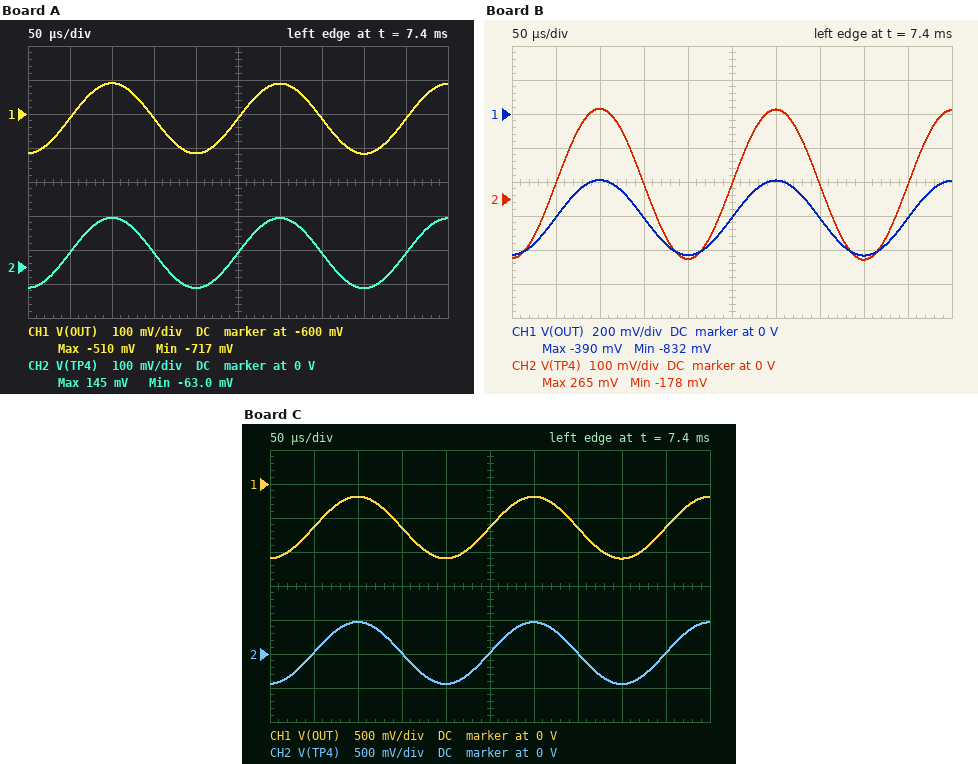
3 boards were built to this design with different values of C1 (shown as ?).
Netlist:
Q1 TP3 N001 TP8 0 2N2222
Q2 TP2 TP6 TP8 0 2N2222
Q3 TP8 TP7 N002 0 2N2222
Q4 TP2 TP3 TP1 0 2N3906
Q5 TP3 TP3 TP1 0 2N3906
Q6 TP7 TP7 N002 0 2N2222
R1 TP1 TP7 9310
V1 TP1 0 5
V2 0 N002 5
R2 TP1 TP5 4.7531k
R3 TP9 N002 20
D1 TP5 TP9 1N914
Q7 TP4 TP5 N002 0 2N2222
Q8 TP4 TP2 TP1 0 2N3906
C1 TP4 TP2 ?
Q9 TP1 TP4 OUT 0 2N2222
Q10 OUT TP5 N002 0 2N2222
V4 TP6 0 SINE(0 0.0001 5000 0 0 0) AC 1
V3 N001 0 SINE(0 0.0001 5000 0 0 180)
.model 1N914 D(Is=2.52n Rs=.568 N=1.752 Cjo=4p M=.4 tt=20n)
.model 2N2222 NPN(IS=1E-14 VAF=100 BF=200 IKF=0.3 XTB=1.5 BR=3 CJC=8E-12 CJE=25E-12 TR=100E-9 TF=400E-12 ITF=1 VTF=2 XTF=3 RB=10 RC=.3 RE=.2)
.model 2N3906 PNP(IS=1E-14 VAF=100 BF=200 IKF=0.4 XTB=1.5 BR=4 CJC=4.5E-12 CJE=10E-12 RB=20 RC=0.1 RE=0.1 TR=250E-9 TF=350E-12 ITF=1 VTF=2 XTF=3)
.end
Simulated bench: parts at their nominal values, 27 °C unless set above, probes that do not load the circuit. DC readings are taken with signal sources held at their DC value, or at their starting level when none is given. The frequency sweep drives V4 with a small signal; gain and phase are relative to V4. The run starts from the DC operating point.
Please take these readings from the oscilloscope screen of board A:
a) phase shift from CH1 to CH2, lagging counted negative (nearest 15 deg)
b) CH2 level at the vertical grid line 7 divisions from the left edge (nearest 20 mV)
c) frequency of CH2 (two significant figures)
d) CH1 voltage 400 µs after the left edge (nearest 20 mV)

0 deg
40 mV
5.0 kHz
-720 mV
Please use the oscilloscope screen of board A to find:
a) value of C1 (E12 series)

1.2 nF
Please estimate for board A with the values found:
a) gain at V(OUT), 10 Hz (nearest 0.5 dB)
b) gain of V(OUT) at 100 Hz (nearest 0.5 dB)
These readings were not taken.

104.0 dB
88.0 dB
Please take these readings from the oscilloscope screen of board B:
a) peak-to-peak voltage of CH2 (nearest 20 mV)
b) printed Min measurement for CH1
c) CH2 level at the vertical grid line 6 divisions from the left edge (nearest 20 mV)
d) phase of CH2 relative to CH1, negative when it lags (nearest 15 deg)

440 mV
-832 mV
260 mV
0 deg
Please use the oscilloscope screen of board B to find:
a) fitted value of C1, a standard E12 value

560 pF
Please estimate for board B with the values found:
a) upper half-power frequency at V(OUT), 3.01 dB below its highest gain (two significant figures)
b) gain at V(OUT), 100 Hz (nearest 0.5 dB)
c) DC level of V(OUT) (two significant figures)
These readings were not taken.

28 Hz
94.5 dB
-670 mV
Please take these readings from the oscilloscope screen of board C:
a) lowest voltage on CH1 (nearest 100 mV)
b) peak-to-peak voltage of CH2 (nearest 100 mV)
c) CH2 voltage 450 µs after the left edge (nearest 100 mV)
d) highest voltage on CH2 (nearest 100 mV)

-1.1 V
900 mV
0 V
500 mV
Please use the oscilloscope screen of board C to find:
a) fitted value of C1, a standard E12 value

270 pF
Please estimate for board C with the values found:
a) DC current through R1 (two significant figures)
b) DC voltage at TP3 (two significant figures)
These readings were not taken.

1.0 mA
4.4 V
